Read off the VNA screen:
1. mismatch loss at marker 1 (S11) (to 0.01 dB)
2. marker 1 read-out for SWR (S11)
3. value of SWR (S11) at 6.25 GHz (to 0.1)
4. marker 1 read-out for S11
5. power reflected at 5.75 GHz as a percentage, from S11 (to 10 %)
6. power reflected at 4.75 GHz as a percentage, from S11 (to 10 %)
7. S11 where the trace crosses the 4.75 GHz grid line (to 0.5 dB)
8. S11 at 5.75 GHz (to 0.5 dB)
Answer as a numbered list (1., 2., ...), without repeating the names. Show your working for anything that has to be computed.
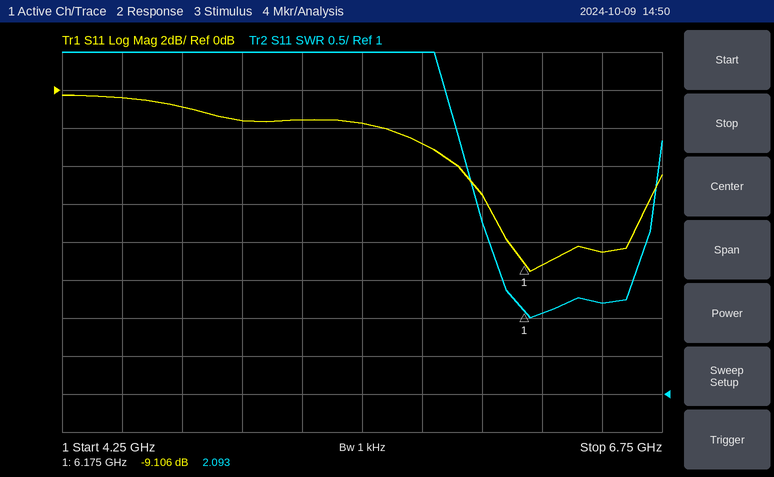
1. −10 log10(1 − 10^(-9.106/10)) ≈ 0.57 dB
2. 2.093
3. 2.1
4. -9.106 dB
5. 10^(-3/10) ≈ 50 %
6. 10^(-1/10) ≈ 79.4 %, so 80 % to the nearest 10 %
7. -1.0 dB
8. -3.0 dB
